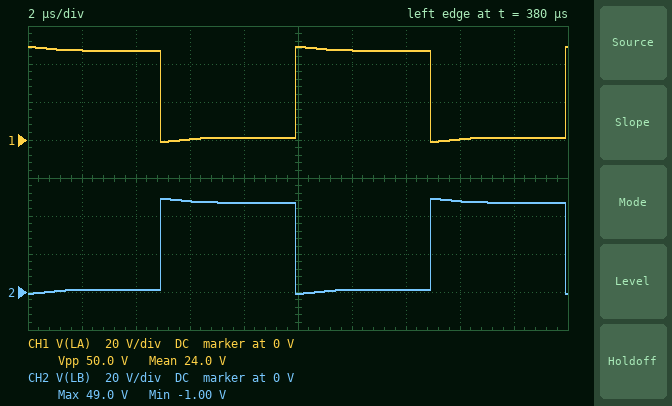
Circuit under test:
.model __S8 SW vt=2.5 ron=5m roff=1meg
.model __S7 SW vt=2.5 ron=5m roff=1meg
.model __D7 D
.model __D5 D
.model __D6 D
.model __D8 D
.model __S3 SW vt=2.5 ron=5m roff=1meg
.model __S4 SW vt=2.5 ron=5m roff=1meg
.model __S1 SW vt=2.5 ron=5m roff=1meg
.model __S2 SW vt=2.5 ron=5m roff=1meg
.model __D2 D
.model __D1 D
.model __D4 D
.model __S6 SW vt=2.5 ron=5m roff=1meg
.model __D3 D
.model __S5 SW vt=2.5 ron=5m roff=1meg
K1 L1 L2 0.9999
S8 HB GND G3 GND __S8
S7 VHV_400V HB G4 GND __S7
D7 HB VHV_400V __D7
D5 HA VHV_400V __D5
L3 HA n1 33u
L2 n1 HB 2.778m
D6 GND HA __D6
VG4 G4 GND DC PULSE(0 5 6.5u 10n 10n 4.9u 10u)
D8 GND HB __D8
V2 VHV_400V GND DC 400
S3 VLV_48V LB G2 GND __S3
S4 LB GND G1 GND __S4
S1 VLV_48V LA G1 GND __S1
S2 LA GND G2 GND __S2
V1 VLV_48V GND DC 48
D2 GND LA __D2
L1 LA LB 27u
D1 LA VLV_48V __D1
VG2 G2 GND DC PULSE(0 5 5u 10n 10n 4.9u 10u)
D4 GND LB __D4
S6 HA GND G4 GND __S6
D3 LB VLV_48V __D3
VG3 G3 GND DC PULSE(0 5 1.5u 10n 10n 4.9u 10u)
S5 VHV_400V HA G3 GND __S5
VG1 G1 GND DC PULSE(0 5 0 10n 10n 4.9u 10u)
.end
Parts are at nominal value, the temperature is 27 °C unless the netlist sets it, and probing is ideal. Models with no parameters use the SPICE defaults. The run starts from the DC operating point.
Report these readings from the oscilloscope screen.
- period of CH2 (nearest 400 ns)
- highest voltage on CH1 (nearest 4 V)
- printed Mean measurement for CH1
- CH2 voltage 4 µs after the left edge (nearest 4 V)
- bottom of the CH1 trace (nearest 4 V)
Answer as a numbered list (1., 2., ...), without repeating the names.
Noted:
1. 10.0 µs
2. 48 V
3. 24.0 V
4. 0 V
5. 0 V
